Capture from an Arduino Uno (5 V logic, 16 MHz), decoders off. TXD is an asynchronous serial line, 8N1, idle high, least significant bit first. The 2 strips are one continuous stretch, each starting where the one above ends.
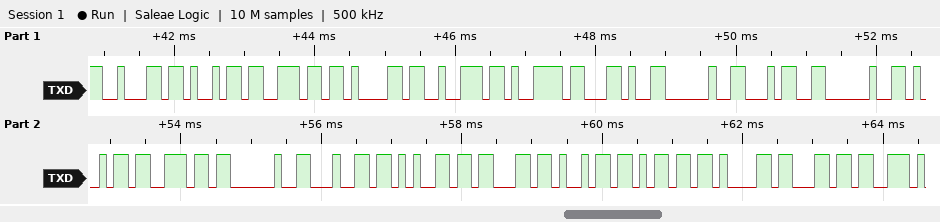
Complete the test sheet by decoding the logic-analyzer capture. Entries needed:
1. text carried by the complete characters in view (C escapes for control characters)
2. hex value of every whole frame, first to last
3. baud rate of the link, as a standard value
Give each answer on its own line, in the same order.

"binary, 4 in decimal"
62 69 6E 61 72 79 2C 20 34 20 69 6E 20 64 65 63 69 6D 61 6C
9600 baud
